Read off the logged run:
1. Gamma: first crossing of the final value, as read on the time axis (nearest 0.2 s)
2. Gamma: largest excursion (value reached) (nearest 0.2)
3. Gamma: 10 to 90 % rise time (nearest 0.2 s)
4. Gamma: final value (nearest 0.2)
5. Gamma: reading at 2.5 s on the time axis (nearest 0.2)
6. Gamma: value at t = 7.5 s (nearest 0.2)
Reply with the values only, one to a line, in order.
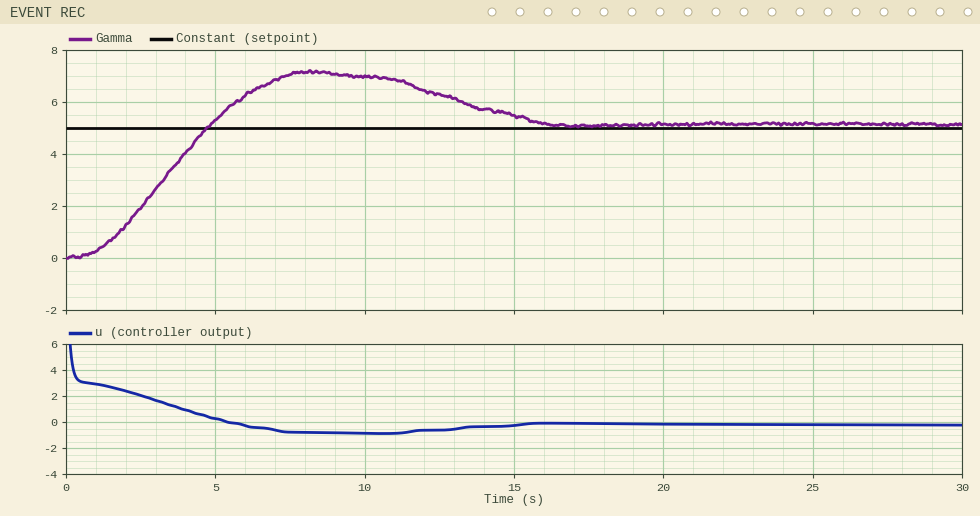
4.8 s
7.2
3.2 s
5.2
2.0
7.0
